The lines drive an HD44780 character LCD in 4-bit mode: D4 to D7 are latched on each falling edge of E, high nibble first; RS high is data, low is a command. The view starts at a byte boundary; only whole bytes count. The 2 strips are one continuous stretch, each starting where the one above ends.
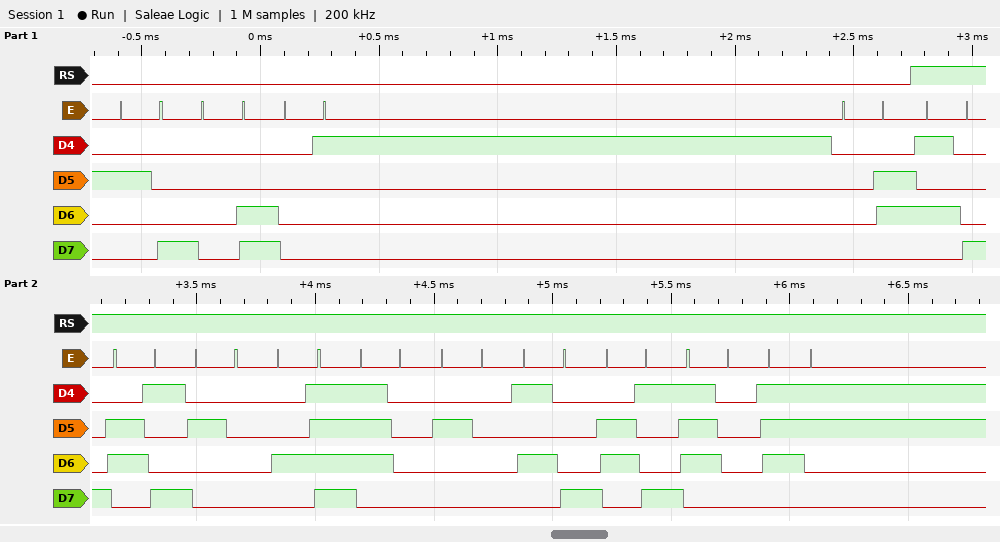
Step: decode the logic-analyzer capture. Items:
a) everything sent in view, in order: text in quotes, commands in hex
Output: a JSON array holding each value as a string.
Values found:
["0x28 0x0C 0x01 0x06 \"Xi Op Xips\""]
